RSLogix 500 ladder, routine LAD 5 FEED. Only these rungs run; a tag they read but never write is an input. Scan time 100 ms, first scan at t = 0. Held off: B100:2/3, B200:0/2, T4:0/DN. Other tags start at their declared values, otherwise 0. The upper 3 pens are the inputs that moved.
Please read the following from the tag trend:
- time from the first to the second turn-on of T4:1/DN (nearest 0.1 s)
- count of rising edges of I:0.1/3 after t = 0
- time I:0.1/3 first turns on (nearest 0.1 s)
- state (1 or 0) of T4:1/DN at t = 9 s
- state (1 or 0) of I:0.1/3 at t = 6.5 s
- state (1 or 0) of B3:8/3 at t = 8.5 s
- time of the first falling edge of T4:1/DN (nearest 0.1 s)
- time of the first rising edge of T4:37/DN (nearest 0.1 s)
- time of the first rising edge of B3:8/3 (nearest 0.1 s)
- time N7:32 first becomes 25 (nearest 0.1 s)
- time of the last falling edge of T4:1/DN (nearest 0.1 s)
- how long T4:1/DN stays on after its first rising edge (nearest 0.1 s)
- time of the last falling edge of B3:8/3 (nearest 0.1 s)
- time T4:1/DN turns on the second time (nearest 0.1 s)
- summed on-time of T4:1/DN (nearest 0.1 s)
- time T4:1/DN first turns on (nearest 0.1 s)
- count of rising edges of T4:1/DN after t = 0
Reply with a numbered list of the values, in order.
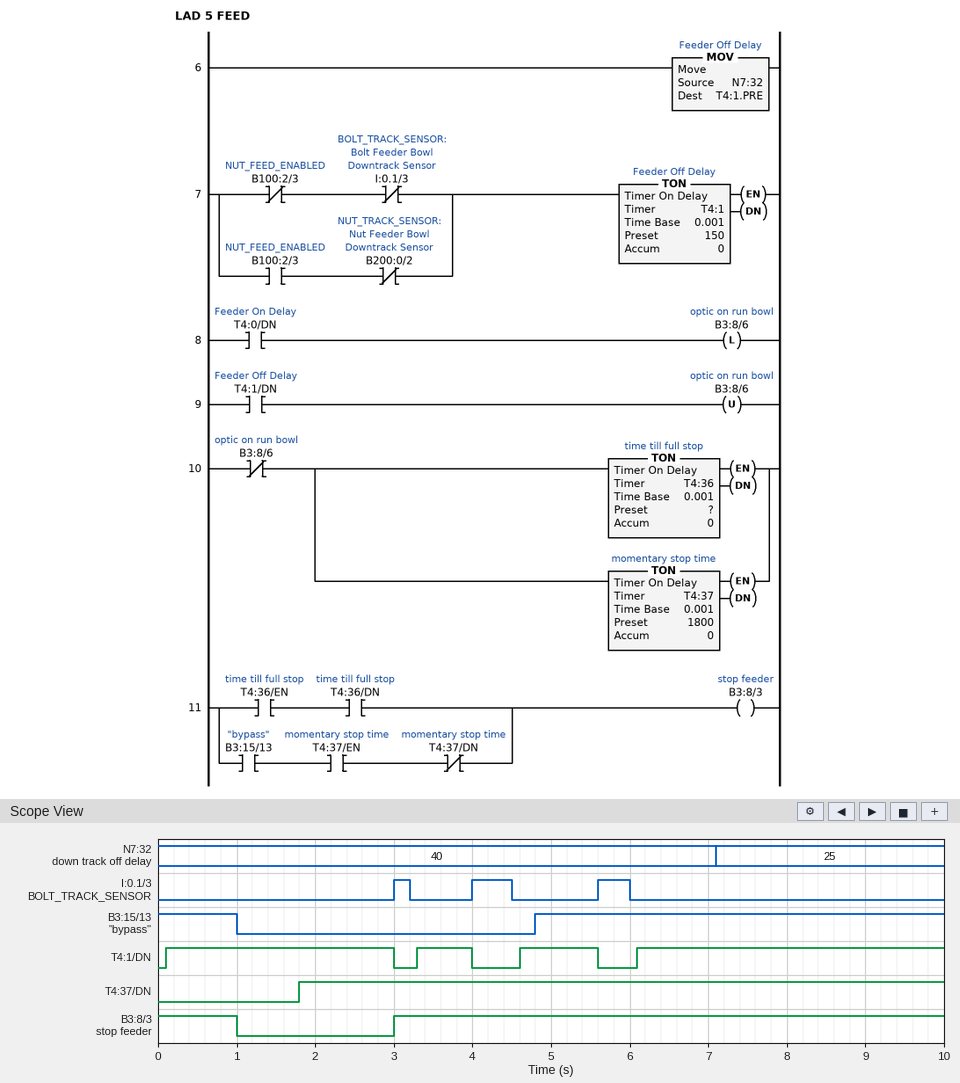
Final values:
1. 3.2 s
2. 3
3. 3.0 s
4. 1
5. 0
6. 1
7. 3.0 s
8. 1.8 s
9. 3.0 s
10. 7.1 s
11. 5.6 s
12. 2.9 s
13. 1.0 s
14. 3.3 s
15. 8.5 s
16. 0.1 s
17. 4
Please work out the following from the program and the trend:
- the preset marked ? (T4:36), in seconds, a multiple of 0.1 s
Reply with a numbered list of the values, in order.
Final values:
1. 3.0 s
